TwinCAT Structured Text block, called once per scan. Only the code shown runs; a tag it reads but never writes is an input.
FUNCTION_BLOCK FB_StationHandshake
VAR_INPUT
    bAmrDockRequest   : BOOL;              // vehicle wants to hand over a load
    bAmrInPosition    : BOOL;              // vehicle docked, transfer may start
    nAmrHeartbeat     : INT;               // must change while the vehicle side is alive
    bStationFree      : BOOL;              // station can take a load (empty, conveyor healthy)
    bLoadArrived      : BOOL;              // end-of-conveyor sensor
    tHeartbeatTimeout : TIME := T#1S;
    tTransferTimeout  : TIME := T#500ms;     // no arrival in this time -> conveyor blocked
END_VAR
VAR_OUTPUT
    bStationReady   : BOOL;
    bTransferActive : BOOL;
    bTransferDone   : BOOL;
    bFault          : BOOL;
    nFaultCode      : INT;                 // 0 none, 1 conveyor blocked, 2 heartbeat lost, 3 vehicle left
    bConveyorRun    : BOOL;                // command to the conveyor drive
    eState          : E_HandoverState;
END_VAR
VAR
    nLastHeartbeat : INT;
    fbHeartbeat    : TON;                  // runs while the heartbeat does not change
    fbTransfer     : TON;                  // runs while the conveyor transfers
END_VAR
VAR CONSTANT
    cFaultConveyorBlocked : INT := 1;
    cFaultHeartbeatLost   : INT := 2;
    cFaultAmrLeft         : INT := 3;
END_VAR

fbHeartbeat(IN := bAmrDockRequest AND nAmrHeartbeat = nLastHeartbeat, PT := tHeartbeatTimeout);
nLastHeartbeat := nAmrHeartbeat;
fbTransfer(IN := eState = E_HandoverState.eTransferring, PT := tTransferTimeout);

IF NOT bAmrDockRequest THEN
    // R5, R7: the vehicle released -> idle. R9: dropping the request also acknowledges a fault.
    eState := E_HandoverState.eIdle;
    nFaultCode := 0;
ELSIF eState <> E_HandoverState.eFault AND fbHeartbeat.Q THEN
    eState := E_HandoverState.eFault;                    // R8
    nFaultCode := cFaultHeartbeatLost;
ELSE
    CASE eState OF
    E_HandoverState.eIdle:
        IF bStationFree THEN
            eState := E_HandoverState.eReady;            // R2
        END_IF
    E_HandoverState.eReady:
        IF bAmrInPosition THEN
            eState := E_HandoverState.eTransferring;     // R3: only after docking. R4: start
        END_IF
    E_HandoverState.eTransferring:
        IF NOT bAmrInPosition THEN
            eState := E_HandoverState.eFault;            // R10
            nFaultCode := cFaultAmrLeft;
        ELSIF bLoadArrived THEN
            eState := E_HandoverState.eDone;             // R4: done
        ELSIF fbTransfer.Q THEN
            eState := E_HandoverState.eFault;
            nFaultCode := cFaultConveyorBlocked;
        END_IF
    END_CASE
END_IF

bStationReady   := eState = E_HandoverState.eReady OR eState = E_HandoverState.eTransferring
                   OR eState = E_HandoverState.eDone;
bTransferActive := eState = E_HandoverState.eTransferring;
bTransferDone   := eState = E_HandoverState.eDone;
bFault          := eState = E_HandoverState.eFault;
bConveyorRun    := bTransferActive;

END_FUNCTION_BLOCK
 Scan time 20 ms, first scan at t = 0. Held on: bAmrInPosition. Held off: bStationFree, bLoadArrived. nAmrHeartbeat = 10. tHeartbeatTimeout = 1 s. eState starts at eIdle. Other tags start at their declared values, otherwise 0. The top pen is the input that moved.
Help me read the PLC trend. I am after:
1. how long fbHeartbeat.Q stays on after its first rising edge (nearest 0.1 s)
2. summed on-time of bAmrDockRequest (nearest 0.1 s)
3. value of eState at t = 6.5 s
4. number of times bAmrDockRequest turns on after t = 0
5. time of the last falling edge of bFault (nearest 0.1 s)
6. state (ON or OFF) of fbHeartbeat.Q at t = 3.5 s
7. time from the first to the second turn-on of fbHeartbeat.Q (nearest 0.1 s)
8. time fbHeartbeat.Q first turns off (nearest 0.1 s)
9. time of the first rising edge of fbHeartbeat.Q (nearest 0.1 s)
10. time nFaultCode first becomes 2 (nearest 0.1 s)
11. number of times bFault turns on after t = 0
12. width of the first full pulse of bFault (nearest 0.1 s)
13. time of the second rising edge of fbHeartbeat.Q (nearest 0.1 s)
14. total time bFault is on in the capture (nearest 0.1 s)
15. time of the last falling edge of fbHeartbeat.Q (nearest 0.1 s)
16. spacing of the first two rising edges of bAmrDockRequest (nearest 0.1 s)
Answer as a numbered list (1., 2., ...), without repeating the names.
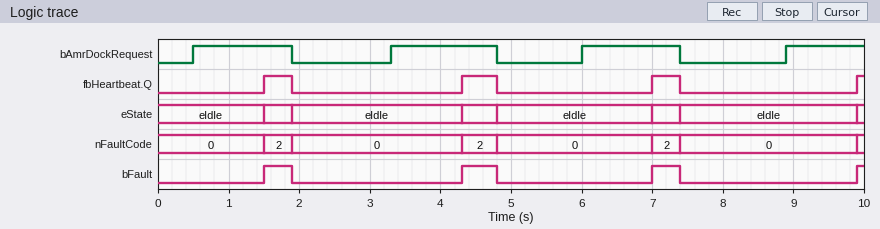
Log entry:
1. 0.4 s
2. 5.4 s
3. eIdle
4. 4
5. 7.4 s
6. OFF
7. 2.8 s
8. 1.9 s
9. 1.5 s
10. 1.5 s
11. 4
12. 0.4 s
13. 4.3 s
14. 1.4 s
15. 7.4 s
16. 2.8 s
